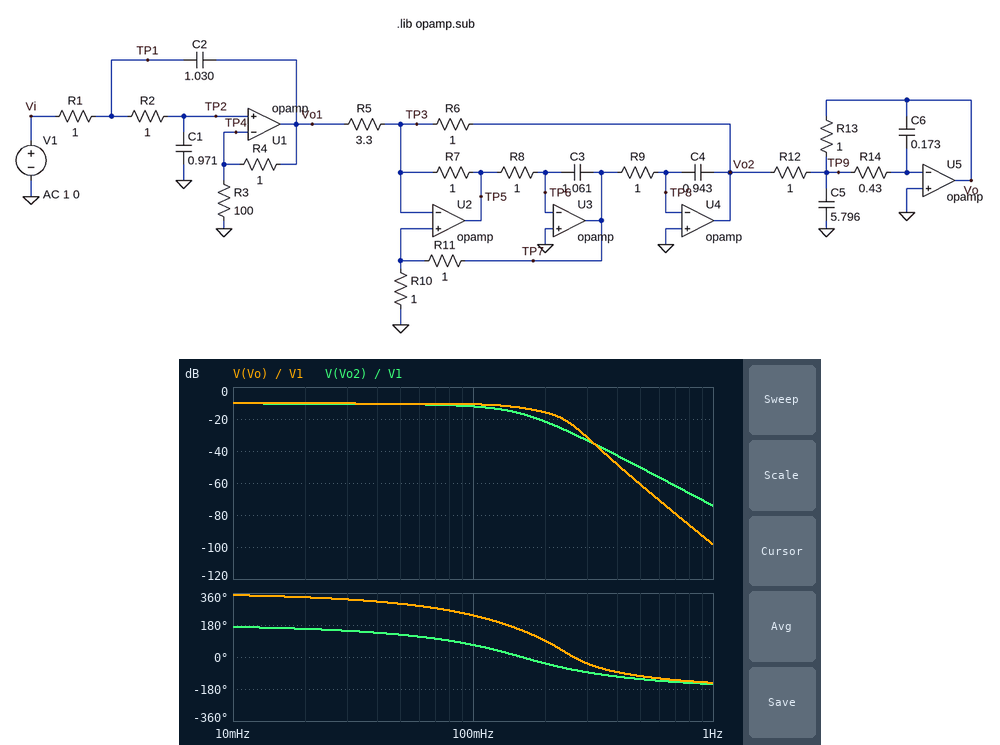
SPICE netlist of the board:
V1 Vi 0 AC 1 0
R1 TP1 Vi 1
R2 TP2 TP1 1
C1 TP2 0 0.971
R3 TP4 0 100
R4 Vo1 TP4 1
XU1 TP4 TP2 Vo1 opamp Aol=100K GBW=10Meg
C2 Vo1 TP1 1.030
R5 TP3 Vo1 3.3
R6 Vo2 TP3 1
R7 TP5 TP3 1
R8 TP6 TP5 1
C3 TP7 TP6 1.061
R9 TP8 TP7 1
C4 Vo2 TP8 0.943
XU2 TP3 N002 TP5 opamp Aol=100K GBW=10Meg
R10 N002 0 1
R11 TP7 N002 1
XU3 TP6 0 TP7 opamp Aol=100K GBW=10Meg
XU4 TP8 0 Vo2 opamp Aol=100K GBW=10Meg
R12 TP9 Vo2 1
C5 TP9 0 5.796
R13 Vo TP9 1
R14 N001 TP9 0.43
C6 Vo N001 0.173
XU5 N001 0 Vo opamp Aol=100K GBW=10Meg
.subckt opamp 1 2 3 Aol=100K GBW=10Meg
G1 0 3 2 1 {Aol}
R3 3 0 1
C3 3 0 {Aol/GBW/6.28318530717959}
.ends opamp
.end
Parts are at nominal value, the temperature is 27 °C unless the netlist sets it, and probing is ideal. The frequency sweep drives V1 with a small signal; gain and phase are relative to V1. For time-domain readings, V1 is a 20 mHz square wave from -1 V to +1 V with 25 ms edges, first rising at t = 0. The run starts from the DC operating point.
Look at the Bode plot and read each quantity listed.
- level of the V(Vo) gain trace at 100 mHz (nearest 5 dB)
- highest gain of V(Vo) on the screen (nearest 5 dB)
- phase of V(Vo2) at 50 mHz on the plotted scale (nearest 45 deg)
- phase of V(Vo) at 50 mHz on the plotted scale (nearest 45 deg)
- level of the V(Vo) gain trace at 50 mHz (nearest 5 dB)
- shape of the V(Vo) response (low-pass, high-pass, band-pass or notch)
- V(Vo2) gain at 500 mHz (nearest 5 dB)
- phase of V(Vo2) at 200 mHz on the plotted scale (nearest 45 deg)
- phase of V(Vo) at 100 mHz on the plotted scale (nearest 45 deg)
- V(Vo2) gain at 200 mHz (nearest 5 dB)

-10 dB
-10 dB
135 deg
315 deg
-10 dB
low-pass
-50 dB
-45 deg
225 deg
-20 dB
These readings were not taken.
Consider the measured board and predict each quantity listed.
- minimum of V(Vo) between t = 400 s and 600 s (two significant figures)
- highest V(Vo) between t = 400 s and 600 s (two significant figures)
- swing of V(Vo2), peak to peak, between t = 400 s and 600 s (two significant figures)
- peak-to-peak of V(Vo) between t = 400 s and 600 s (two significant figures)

-360 mV
360 mV
650 mV
720 mV
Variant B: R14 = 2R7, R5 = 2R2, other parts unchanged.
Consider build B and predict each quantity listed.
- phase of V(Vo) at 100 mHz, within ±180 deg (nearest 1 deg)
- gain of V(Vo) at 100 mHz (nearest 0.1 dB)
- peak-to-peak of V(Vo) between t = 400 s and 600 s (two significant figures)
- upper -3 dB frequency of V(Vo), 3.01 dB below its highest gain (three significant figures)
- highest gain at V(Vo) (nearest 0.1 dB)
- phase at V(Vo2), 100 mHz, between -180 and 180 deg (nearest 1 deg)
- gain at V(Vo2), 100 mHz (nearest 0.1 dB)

151 deg
-5.8 dB
1.4 V
107 mHz
-4.2 dB
66 deg
-8.9 dB
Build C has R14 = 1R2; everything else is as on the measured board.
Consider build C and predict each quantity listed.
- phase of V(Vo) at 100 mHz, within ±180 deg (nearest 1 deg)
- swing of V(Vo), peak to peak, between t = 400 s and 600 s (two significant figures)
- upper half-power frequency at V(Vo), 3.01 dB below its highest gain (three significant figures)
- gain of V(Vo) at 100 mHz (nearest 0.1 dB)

-147 deg
930 mV
151 mHz
-8.3 dB
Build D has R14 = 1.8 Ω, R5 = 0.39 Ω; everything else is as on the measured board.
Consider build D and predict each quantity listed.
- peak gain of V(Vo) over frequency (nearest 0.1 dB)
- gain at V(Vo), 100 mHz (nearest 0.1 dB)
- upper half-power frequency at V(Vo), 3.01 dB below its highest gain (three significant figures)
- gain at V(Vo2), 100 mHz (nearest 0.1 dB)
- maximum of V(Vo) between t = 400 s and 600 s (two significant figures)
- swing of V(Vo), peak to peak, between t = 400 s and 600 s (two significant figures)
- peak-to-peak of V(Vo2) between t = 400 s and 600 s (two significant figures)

8.3 dB
7.0 dB
116 mHz
2.2 dB
3.1 V
6.1 V
5.2 V
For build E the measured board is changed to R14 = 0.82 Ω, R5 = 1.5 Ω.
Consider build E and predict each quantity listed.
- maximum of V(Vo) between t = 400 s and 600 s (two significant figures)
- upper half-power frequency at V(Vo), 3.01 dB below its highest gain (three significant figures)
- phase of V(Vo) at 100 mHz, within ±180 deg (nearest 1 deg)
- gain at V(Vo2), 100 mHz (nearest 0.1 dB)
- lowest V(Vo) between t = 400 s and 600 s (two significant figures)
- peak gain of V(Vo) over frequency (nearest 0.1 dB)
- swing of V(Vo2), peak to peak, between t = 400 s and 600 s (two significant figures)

880 mV
171 mHz
-139 deg
-6.0 dB
-880 mV
-3.3 dB
1.4 V
